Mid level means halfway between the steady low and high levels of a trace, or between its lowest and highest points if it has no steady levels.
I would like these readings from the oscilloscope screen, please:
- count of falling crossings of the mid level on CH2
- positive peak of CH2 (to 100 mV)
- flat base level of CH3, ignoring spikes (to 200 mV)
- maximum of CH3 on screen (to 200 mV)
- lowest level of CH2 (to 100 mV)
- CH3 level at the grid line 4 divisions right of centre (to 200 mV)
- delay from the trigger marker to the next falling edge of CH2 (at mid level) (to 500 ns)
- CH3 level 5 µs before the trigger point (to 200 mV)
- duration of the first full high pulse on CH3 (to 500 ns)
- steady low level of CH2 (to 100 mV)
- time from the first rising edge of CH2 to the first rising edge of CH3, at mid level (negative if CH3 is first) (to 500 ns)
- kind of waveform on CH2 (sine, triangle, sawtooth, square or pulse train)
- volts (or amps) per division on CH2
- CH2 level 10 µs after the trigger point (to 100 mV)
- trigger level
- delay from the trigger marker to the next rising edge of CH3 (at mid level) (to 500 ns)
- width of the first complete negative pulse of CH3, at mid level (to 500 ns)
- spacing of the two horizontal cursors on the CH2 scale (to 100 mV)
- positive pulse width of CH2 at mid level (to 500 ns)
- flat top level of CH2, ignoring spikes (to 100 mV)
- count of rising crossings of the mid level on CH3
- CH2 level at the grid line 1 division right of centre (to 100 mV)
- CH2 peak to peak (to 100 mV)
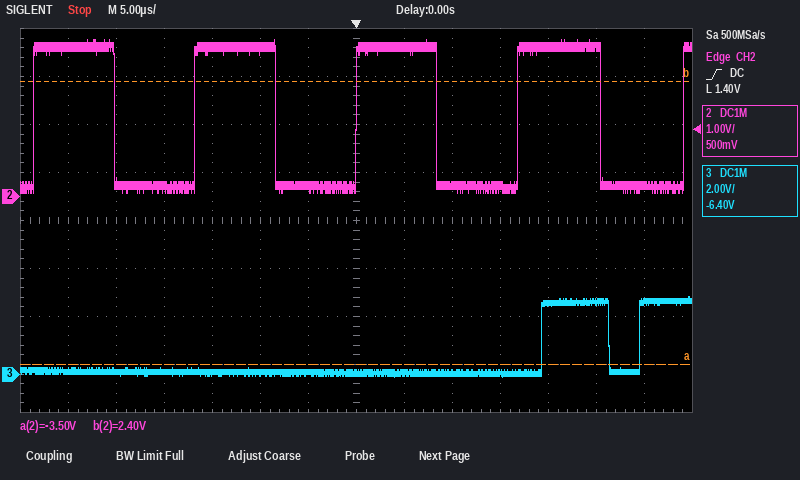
4
3.3 V
200 mV
3.2 V
100 mV
3.0 V
8.5 µs
200 mV
7.0 µs
200 mV
+53.0 µs
square
1 V
200 mV
1.40 V
19.5 µs
3.0 µs
5.9 V
8.5 µs
3.1 V
2
3.1 V
3.2 V
